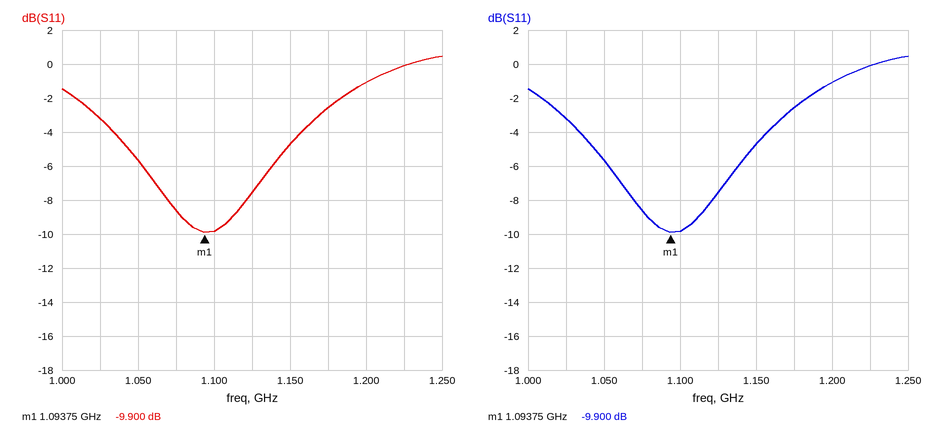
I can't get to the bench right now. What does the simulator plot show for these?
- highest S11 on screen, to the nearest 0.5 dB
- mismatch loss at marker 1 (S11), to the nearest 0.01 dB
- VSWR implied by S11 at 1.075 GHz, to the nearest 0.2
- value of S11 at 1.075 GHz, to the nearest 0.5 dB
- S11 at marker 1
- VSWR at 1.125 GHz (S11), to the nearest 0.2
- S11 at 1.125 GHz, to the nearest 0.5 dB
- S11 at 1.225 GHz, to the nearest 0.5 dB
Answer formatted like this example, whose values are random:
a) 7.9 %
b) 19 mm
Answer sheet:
a) 0.5 dB
b) 0.47 dB
c) 2.2
d) -8.5 dB
e) -9.900 dB
f) 2.4
g) -7.5 dB
h) 0.0 dB
